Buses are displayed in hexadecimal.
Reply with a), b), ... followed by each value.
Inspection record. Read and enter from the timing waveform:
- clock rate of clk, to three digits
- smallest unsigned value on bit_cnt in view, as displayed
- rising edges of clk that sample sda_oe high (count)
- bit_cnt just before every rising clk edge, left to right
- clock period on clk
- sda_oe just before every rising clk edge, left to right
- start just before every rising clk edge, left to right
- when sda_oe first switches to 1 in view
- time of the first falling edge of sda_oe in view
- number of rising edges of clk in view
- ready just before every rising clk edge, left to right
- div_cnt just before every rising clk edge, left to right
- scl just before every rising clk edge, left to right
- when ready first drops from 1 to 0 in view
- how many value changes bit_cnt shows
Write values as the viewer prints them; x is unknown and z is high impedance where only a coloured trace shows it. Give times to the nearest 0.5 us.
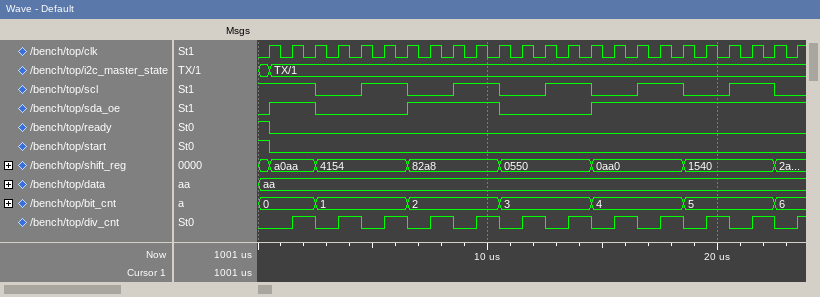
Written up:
a) 1.00 MHz
b) 0
c) 15
d) 0, 0, 0, 1, 1, 1, 1, 2, 2, 2, 2, 3, 3, 3, 3, 4, 4, 4, 4, 5, 5, 5, 5, 6
e) 1 us
f) 0 1 1 0 0 0 0 1 1 1 1 0 0 0 0 1 1 1 1 1 1 1 1 1
g) 1 0 0 0 0 0 0 0 0 0 0 0 0 0 0 0 0 0 0 0 0 0 0 0
h) 0.5 us
i) 2.5 us
j) 24
k) 1 0 0 0 0 0 0 0 0 0 0 0 0 0 0 0 0 0 0 0 0 0 0 0
l) 0 0 1 0 1 0 1 0 1 0 1 0 1 0 1 0 1 0 1 0 1 0 1 0
m) 1 1 1 0 0 1 1 0 0 1 1 0 0 1 1 0 0 1 1 0 0 1 1 0
n) 0.5 us
o) 6
